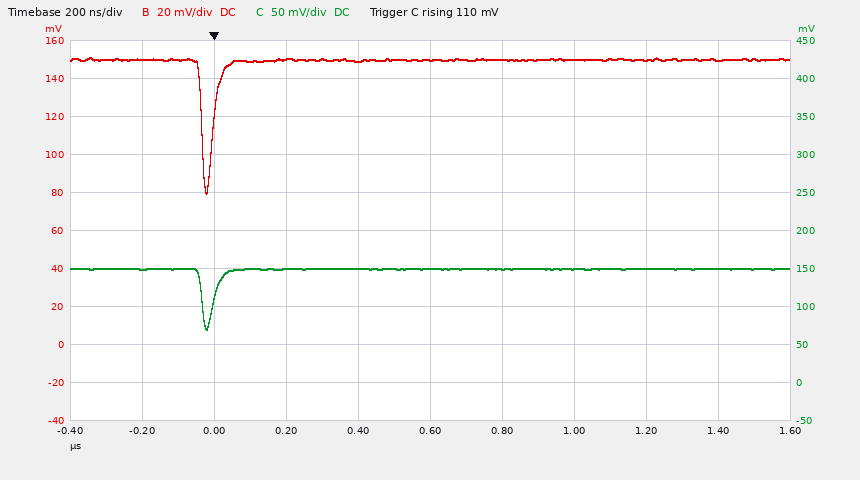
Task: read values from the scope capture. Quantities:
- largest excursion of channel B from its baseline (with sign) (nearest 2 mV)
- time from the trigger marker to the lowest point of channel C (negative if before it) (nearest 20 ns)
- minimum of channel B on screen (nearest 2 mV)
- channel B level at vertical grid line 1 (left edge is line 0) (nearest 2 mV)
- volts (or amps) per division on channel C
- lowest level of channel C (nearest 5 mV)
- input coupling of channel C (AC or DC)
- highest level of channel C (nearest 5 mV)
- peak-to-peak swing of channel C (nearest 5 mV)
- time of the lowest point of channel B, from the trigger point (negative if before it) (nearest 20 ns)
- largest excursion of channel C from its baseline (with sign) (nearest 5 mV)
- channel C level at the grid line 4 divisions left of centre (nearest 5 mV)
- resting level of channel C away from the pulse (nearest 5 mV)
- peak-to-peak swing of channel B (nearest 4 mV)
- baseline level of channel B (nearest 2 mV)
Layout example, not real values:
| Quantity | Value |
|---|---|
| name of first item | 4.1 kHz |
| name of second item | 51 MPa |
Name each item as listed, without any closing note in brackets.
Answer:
| Quantity | Value |
|---|---|
| largest excursion of channel B from its baseline (with sign) | -70 mV |
| time from the trigger marker to the lowest point of channel C (negative if before it) | -20 ns |
| minimum of channel B on screen | 80 mV |
| channel B level at vertical grid line 1 (left edge is line 0) | 150 mV |
| volts (or amps) per division on channel C | 50 mV |
| lowest level of channel C | 70 mV |
| input coupling of channel C | DC |
| highest level of channel C | 150 mV |
| peak-to-peak swing of channel C | 80 mV |
| time of the lowest point of channel B, from the trigger point (negative if before it) | -20 ns |
| largest excursion of channel C from its baseline (with sign) | -80 mV |
| channel C level at the grid line 4 divisions left of centre | 150 mV |
| resting level of channel C away from the pulse | 150 mV |
| peak-to-peak swing of channel B | 72 mV |
| baseline level of channel B | 150 mV |
